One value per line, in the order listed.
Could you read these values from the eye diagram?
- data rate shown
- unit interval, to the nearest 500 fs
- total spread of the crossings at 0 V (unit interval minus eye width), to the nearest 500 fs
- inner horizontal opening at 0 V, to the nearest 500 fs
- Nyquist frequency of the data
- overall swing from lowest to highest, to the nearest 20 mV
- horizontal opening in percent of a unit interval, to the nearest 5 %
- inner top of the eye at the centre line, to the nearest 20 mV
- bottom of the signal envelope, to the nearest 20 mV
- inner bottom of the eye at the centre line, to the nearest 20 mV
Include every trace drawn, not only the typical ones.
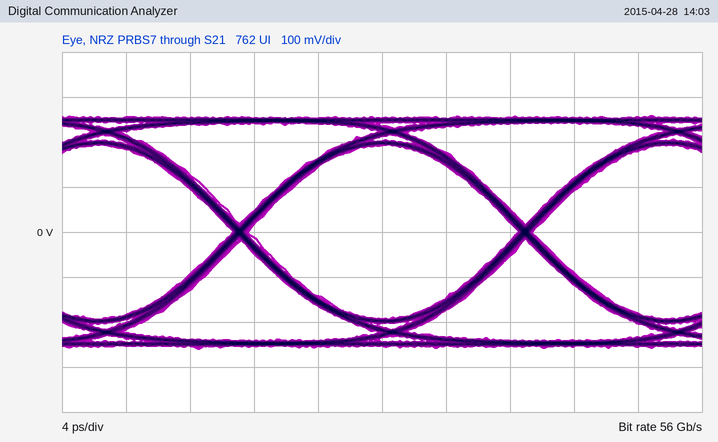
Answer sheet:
56 Gb/s
18.0 ps
1.0 ps
17.0 ps
28 GHz
520 mV
95 %
200 mV
-260 mV
-200 mV
